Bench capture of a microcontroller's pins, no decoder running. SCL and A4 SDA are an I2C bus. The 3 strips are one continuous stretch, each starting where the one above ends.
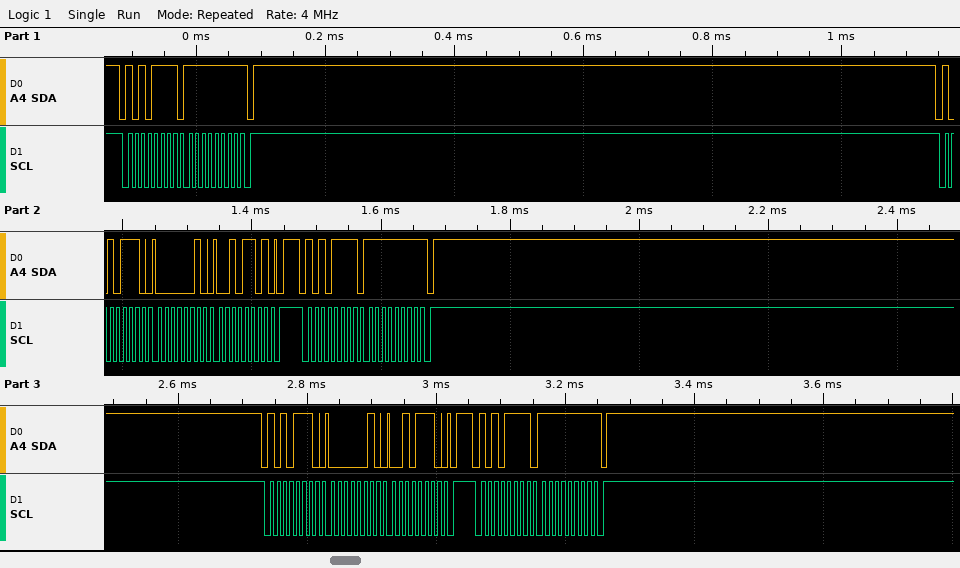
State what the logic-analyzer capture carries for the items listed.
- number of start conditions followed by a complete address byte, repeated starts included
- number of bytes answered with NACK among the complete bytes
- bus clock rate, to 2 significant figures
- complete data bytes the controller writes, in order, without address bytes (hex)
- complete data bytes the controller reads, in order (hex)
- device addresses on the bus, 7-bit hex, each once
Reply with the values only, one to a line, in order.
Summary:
5
3
100 kHz
02 2D 02 2E
FF FF FF
0x57
